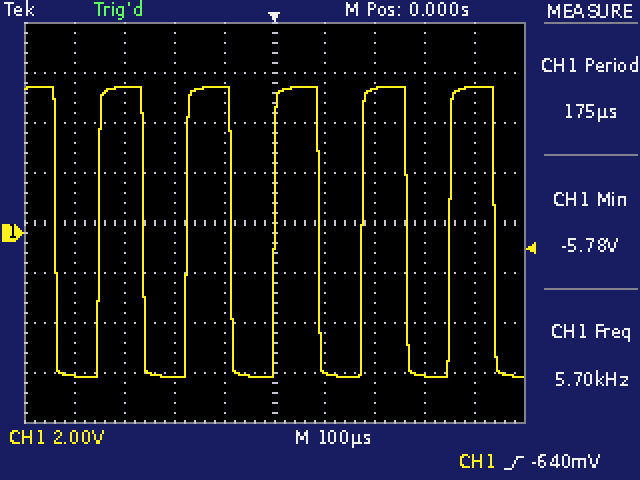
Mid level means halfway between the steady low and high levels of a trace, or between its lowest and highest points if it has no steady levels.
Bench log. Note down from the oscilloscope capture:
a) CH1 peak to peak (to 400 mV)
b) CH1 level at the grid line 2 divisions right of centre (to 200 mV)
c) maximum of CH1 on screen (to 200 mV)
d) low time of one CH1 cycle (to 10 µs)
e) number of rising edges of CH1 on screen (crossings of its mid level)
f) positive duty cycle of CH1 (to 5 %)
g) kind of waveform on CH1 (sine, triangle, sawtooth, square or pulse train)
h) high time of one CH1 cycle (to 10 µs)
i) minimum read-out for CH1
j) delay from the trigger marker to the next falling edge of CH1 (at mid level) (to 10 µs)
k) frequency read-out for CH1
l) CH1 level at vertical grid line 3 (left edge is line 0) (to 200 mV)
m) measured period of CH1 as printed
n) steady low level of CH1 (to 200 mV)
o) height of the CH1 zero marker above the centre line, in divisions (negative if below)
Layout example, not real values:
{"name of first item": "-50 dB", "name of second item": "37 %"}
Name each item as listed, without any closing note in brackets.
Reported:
{"CH1 peak to peak": "11.6 V", "CH1 level at the grid line 2 divisions right of centre": "5.8 V", "maximum of CH1 on screen": "5.8 V", "low time of one CH1 cycle": "90 µs", "number of rising edges of CH1 on screen": "5", "positive duty cycle of CH1": "50 %", "kind of waveform on CH1": "square", "high time of one CH1 cycle": "90 µs", "minimum read-out for CH1": "-5.78 V", "delay from the trigger marker to the next falling edge of CH1 (at mid level)": "90 µs", "frequency read-out for CH1": "5.70 kHz", "CH1 level at vertical grid line 3 (left edge is line 0)": "-5.8 V", "measured period of CH1 as printed": "175 µs", "steady low level of CH1": "-5.8 V", "height of the CH1 zero marker above the centre line, in divisions": "-0.2 div"}
